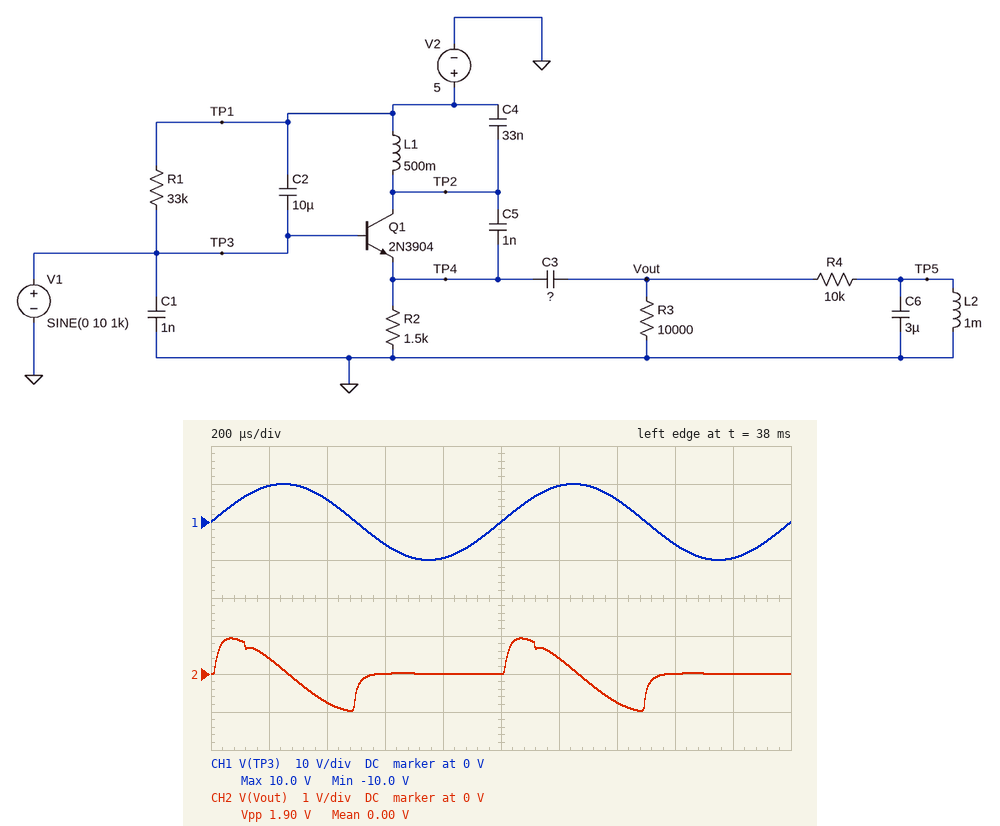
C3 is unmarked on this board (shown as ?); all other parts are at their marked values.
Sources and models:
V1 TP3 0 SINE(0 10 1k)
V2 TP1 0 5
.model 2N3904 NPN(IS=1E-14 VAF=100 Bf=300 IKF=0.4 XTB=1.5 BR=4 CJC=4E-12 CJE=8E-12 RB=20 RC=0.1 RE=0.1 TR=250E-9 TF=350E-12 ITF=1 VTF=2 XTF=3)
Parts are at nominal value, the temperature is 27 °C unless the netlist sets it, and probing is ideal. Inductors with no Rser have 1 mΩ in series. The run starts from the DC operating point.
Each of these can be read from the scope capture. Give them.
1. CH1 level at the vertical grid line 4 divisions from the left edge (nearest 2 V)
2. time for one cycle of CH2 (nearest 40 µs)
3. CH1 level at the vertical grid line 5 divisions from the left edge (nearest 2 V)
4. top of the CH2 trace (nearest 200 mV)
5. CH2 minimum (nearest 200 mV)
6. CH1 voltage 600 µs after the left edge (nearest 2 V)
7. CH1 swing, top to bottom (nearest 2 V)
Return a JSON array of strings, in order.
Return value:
["-10 V", "1.00 ms", "0 V", "1.0 V", "-1.0 V", "-6 V", "20 V"]
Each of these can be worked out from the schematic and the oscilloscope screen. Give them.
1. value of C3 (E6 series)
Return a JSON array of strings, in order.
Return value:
["3.3 nF"]
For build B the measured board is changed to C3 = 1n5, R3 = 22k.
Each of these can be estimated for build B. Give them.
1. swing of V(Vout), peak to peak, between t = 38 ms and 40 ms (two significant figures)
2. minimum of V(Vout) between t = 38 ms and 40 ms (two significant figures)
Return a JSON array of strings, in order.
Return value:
["1.2 V", "-610 mV"]
